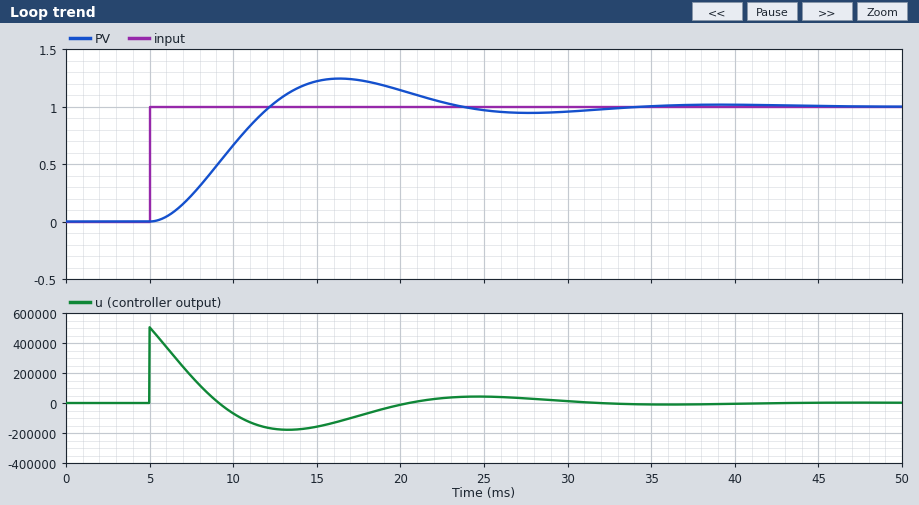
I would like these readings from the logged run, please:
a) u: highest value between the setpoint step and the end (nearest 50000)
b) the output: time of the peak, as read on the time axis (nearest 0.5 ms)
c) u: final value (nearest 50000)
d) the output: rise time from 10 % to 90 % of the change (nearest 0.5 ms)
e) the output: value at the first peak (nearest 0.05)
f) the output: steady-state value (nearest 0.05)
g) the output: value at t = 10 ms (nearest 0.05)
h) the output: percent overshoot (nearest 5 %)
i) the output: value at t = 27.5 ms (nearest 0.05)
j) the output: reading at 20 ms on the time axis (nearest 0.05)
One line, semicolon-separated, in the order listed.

500000; 16.5 ms; 0; 5.0 ms; 1.25; 1.00; 0.65; 25 %; 0.95; 1.15
